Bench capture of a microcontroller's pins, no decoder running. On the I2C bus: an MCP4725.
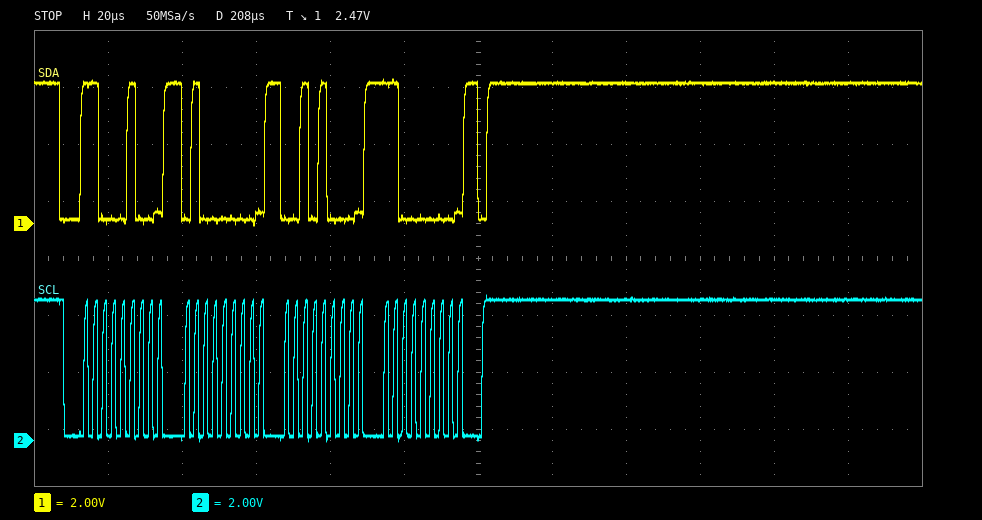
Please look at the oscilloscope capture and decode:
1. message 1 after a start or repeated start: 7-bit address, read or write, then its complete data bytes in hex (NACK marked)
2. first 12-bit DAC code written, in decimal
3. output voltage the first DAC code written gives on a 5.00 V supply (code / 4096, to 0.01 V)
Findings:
0x62 write: 40 28 C0
652
0.80 V
